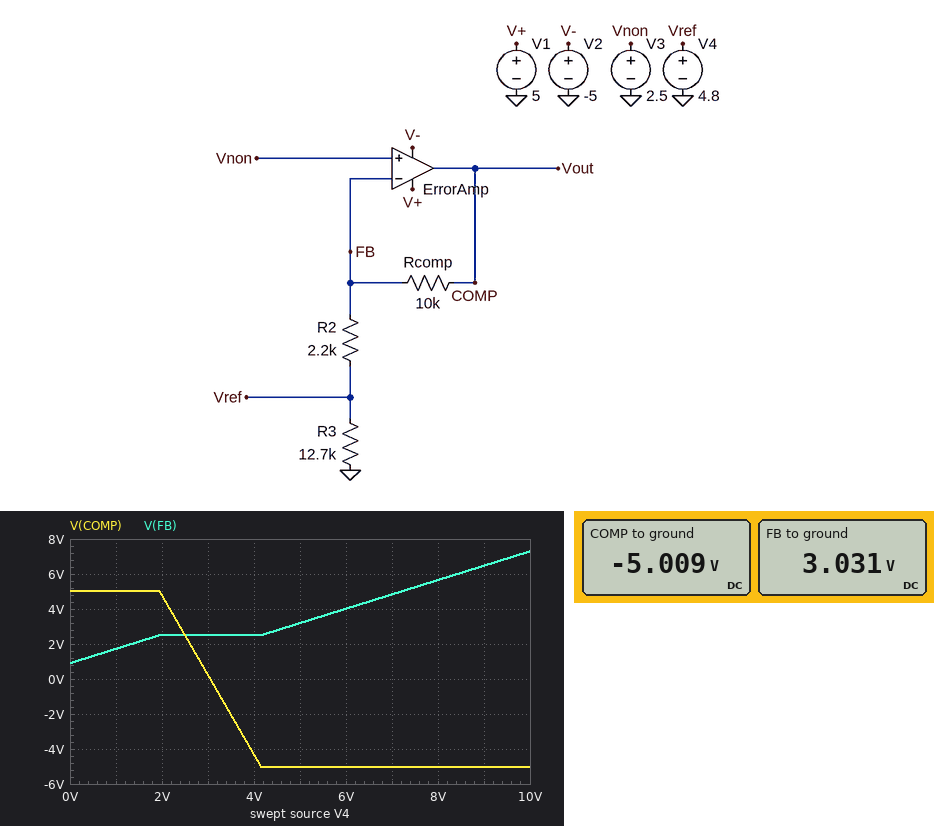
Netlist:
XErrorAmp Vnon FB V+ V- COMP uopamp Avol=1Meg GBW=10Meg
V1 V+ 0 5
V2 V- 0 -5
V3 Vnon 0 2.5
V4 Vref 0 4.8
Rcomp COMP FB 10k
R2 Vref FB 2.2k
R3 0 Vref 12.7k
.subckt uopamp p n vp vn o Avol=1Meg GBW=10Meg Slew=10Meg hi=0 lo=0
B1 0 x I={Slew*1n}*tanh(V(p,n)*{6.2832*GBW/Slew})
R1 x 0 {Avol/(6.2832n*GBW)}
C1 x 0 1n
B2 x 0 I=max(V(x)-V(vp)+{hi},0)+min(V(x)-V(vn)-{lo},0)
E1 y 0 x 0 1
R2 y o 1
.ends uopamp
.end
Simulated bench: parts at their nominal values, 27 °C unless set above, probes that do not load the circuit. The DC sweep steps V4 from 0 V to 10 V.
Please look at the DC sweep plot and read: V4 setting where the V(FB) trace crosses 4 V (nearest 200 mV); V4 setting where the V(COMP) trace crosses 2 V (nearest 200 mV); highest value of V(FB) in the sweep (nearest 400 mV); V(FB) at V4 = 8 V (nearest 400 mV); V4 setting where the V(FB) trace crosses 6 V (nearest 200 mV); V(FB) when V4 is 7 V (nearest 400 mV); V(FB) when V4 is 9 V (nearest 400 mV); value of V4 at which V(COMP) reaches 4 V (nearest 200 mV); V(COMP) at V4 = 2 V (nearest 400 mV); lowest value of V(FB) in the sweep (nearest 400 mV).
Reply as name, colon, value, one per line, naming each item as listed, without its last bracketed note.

V4 setting where the V(FB) trace crosses 4 V: 6.0 V
V4 setting where the V(COMP) trace crosses 2 V: 2.6 V
highest value of V(FB) in the sweep: 7.2 V
V(FB) at V4 = 8 V: 5.6 V
V4 setting where the V(FB) trace crosses 6 V: 8.4 V
V(FB) when V4 is 7 V: 4.8 V
V(FB) when V4 is 9 V: 6.4 V
value of V4 at which V(COMP) reaches 4 V: 2.2 V
V(COMP) at V4 = 2 V: 4.8 V
lowest value of V(FB) in the sweep: 800 mV
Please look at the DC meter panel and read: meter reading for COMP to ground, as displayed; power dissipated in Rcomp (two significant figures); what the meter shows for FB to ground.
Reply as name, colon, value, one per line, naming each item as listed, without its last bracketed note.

meter reading for COMP to ground, as displayed: -5.009 V
power dissipated in Rcomp: 6.5 mW
what the meter shows for FB to ground: 3.031 V
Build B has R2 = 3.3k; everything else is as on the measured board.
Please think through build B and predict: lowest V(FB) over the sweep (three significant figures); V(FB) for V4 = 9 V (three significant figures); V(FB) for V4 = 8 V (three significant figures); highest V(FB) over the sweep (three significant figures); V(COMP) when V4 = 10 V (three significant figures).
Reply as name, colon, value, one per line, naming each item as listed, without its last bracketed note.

lowest V(FB) over the sweep: 1.24 V
V(FB) for V4 = 9 V: 5.52 V
V(FB) for V4 = 8 V: 4.77 V
highest V(FB) over the sweep: 6.28 V
V(COMP) when V4 = 10 V: -5.01 V
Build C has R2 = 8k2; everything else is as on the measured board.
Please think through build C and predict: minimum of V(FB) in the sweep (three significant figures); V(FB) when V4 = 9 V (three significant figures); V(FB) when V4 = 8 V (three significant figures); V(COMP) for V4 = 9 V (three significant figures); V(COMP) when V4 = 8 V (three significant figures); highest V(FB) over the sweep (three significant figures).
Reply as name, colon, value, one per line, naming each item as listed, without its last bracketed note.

minimum of V(FB) in the sweep: 2.26 V
V(FB) when V4 = 9 V: 2.69 V
V(FB) when V4 = 8 V: 2.50 V
V(COMP) for V4 = 9 V: -5.01 V
V(COMP) when V4 = 8 V: -4.21 V
highest V(FB) over the sweep: 3.24 V
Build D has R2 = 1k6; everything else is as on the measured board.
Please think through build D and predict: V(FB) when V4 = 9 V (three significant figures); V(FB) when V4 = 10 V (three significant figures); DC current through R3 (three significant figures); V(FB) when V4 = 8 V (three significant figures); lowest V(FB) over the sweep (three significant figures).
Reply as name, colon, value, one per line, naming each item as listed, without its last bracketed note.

V(FB) when V4 = 9 V: 7.07 V
V(FB) when V4 = 10 V: 7.93 V
DC current through R3: 378 µA
V(FB) when V4 = 8 V: 6.21 V
lowest V(FB) over the sweep: 691 mV
